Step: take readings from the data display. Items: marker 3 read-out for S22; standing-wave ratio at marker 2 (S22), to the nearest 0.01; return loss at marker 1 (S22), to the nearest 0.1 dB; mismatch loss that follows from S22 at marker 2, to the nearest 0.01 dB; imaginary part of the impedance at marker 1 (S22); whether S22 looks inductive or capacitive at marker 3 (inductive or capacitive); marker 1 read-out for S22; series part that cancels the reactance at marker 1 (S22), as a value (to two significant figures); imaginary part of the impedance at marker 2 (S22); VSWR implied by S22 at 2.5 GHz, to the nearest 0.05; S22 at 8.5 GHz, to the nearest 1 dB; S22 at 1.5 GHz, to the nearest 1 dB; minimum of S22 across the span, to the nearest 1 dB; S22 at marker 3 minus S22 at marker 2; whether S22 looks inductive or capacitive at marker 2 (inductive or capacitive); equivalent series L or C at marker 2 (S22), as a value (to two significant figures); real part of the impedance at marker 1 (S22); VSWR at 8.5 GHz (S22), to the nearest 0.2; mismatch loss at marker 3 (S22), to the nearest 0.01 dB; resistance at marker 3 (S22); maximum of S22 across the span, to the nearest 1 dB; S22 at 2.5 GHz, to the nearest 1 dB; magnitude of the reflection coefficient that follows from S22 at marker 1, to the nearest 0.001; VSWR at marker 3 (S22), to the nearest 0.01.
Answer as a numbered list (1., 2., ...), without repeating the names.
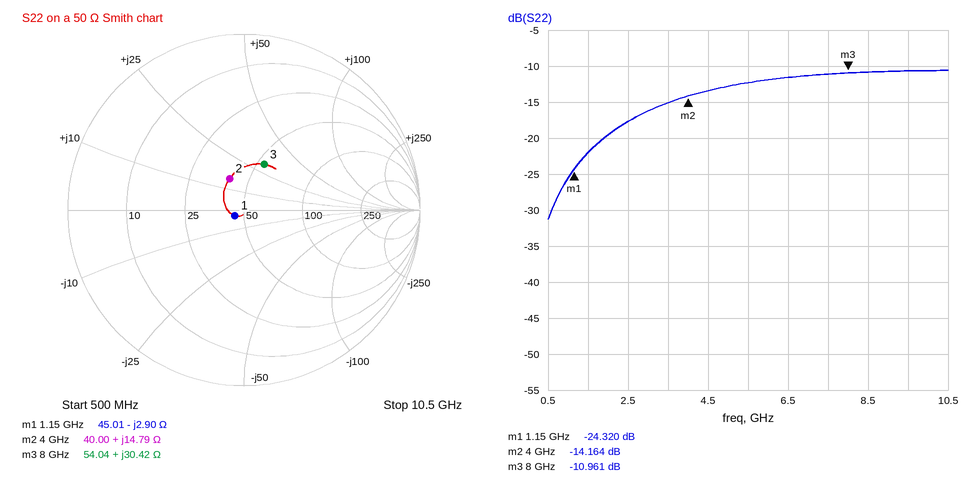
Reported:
1. -10.961 dB
2. 1.49
3. 24.3 dB
4. 0.17 dB
5. -2.90 Ω
6. inductive
7. -24.320 dB
8. 400 pH
9. +14.79 Ω
10. 1.30
11. -11 dB
12. -22 dB
13. -31 dB
14. 3.203 dB
15. inductive
16. 590 pH
17. 45.01 Ω
18. 1.8
19. 0.36 dB
20. 54.04 Ω
21. -11 dB
22. -18 dB
23. 0.061
24. 1.79
